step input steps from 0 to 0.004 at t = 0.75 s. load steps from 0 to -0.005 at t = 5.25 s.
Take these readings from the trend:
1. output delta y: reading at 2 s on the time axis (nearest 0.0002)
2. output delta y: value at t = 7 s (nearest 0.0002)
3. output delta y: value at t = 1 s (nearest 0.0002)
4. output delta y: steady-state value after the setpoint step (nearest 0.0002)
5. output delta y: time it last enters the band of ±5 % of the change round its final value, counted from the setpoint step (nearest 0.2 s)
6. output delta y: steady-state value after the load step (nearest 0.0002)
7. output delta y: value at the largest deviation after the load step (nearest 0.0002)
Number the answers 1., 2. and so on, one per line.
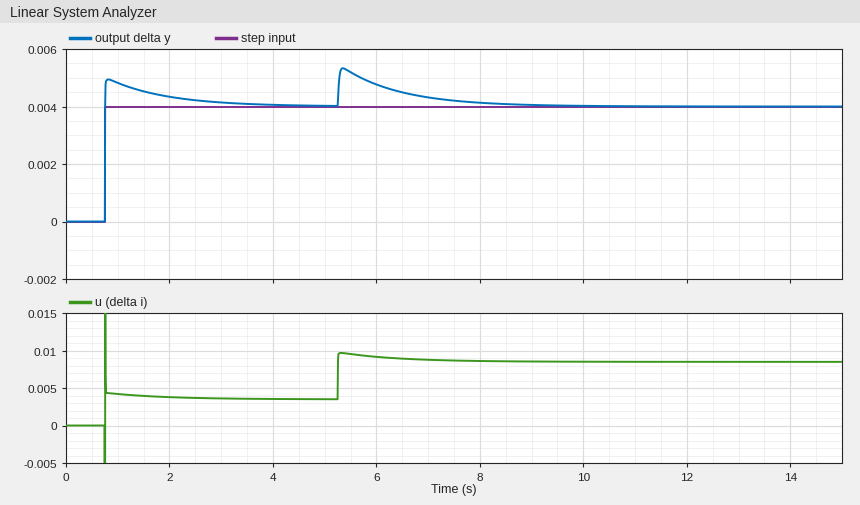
1. 0.0044
2. 0.0044
3. 0.0048
4. 0.0040
5. 1.8 s
6. 0.0040
7. 0.0054
